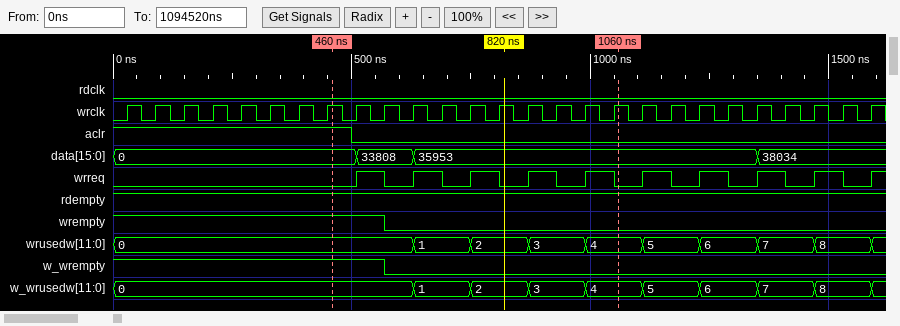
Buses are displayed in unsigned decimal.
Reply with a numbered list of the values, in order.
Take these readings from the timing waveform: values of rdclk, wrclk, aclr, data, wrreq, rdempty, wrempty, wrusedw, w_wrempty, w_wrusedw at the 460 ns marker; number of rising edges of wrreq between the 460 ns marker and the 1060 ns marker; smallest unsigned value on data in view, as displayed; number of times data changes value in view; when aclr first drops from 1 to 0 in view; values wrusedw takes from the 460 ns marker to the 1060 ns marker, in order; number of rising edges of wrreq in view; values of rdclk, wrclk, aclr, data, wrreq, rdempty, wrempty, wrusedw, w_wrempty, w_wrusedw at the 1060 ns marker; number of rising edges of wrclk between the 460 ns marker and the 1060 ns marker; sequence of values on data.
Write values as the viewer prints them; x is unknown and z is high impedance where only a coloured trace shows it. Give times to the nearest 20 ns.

1. rdclk=0, wrclk=1, aclr=1, data=0, wrreq=0, rdempty=1, wrempty=1, wrusedw=0, w_wrempty=1, w_wrusedw=0
2. 5
3. 0
4. 3
5. 500 ns
6. 0, 1, 2, 3, 4
7. 10
8. rdclk=0, wrclk=1, aclr=0, data=35953, wrreq=0, rdempty=1, wrempty=0, wrusedw=4, w_wrempty=0, w_wrusedw=4
9. 10
10. 0, 33808, 35953, 38034
